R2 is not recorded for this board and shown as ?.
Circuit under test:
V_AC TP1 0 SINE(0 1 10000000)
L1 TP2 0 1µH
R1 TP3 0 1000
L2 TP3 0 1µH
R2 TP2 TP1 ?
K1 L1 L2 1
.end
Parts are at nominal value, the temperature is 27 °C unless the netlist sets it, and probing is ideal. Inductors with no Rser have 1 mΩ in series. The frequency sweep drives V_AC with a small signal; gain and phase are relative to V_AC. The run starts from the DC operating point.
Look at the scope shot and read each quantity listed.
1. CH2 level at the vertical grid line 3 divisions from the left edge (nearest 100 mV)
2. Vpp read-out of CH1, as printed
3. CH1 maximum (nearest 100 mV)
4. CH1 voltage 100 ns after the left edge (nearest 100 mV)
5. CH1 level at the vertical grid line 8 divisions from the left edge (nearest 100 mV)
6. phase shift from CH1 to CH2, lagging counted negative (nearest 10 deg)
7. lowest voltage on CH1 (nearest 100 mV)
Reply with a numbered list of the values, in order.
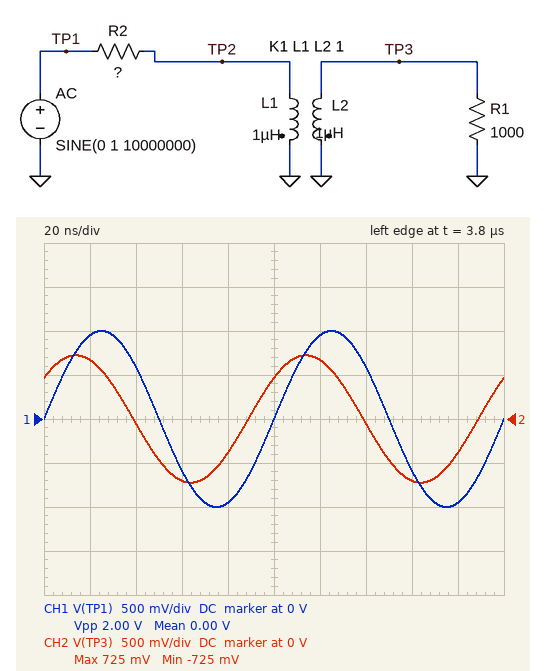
1. -700 mV
2. 2.00 V
3. 1.0 V
4. 0 V
5. -600 mV
6. 40 deg
7. -1.0 V
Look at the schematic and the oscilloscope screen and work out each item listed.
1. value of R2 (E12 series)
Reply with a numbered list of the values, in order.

1. 56 Ω
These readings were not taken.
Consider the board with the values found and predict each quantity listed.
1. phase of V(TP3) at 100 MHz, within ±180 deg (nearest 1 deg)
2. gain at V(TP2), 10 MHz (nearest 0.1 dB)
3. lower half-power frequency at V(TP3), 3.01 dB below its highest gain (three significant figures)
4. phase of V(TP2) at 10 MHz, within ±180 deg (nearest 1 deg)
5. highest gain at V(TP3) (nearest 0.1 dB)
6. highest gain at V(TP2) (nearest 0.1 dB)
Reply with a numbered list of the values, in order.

1. 5 deg
2. -2.8 dB
3. 8.44 MHz
4. 40 deg
5. -0.5 dB
6. -0.5 dB
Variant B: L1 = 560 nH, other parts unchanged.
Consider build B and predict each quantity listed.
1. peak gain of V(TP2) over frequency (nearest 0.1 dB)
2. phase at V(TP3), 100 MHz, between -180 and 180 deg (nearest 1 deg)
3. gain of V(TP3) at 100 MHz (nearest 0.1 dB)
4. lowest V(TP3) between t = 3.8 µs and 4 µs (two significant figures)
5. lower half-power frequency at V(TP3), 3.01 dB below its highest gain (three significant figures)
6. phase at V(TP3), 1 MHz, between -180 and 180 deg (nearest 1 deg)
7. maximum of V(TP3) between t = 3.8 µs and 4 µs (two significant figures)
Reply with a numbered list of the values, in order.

1. -0.8 dB
2. 8 deg
3. 1.6 dB
4. -690 mV
5. 14.5 MHz
6. 86 deg
7. 690 mV
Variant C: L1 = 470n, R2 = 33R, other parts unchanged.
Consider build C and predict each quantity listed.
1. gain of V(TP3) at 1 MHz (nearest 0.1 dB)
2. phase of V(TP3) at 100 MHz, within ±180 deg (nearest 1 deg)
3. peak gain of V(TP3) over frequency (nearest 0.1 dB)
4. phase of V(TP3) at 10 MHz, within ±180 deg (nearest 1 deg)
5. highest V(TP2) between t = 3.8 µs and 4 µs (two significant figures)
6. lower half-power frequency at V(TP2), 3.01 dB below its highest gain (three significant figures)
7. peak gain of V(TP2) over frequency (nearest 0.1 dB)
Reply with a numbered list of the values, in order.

1. -17.7 dB
2. 6 deg
3. 2.7 dB
4. 46 deg
5. 650 mV
6. 10.4 MHz
7. -0.6 dB
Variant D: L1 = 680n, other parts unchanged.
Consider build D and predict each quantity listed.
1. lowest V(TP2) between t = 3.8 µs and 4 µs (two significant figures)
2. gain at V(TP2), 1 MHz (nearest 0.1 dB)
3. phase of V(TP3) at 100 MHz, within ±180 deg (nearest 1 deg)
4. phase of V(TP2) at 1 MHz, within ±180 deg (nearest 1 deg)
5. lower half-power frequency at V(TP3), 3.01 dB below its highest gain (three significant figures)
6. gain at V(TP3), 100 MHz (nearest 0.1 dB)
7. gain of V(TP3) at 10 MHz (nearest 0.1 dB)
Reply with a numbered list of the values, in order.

1. -590 mV
2. -22.4 dB
3. 7 deg
4. 85 deg
5. 12.1 MHz
6. 0.9 dB
7. -2.9 dB
